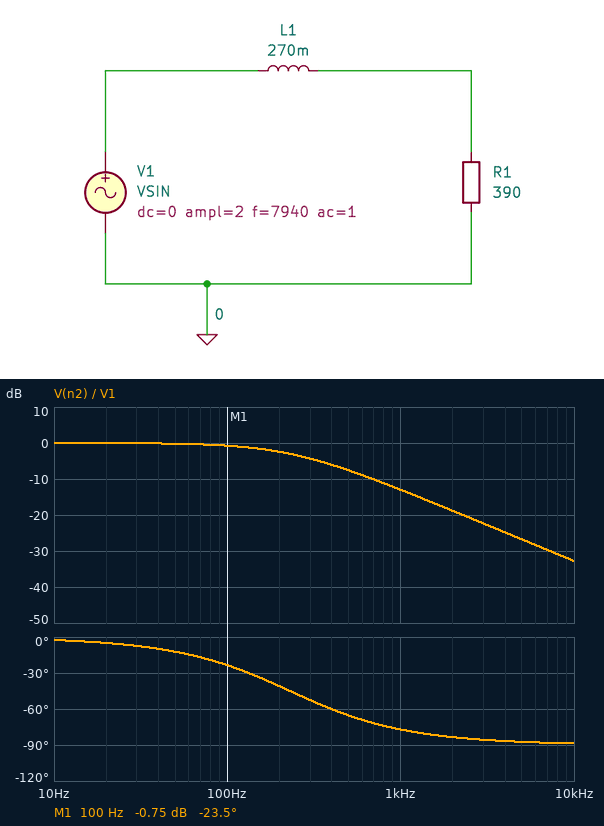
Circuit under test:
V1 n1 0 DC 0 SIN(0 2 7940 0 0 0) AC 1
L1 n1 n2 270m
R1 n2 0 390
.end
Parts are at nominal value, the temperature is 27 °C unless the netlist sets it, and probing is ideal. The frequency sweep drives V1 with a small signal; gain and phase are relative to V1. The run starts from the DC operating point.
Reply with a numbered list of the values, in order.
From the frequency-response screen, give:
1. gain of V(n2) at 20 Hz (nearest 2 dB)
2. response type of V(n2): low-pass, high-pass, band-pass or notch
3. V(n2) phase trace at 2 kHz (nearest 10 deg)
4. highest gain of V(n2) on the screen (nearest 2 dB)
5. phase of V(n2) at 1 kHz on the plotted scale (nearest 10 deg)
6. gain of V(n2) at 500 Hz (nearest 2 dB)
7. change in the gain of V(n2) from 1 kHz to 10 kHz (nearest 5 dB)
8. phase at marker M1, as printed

1. 0 dB
2. low-pass
3. -80 deg
4. 0 dB
5. -80 deg
6. -8 dB
7. -20 dB
8. -23.5 deg
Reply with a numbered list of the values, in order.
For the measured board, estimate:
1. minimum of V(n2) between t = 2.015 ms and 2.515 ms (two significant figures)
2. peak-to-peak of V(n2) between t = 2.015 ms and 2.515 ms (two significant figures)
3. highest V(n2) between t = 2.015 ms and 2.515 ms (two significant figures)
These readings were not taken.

1. -56 mV
2. 120 mV
3. 61 mV
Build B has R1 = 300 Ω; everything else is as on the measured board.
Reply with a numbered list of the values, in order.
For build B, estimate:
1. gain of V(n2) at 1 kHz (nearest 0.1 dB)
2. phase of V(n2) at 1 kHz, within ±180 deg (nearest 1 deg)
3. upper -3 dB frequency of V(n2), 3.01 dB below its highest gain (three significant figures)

1. -15.2 dB
2. -80 deg
3. 177 Hz
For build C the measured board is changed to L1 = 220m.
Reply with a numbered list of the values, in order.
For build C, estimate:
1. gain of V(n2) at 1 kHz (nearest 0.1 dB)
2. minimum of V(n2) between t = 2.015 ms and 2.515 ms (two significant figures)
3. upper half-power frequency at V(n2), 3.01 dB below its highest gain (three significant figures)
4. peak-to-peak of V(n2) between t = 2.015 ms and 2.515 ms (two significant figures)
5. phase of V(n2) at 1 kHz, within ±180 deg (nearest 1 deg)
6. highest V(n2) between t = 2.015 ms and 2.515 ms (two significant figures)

1. -11.3 dB
2. -70 mV
3. 282 Hz
4. 140 mV
5. -74 deg
6. 73 mV
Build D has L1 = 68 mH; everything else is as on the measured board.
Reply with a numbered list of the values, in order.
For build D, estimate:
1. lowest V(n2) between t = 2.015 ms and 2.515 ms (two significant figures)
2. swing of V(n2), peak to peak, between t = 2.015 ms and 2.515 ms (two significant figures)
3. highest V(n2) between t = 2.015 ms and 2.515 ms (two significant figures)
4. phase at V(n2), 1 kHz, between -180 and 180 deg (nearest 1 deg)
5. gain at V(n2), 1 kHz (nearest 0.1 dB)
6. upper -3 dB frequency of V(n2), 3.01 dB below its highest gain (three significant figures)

1. -230 mV
2. 460 mV
3. 230 mV
4. -48 deg
5. -3.4 dB
6. 913 Hz
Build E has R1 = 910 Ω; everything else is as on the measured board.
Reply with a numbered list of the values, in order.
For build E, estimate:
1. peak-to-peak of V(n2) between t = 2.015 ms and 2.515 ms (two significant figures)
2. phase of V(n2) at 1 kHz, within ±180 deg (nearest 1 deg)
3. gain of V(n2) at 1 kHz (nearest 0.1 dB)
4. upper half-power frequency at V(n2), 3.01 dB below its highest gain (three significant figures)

1. 270 mV
2. -62 deg
3. -6.5 dB
4. 536 Hz
